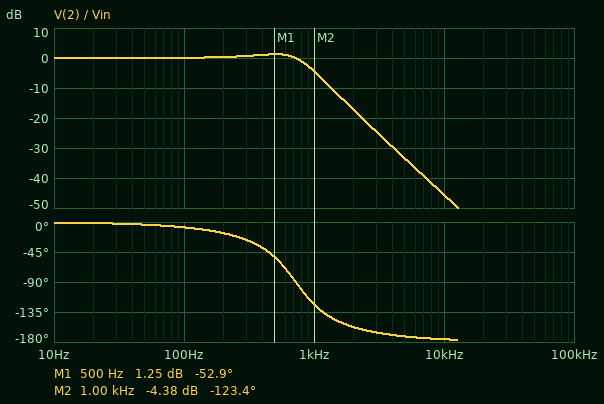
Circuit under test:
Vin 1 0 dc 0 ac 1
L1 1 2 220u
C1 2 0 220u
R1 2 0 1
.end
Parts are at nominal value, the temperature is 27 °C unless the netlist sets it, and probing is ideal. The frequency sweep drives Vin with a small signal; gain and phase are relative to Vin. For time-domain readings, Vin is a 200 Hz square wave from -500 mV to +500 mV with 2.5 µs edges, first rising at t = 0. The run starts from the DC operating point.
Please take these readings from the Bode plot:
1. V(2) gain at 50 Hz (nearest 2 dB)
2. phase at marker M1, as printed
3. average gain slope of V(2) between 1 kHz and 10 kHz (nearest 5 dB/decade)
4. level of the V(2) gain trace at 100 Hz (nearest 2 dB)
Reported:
0 dB
-52.9 deg
-40 dB/decade
0 dB
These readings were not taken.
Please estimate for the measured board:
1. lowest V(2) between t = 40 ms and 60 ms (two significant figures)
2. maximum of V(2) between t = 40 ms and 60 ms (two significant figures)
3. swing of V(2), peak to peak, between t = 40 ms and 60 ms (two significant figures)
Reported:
-660 mV
660 mV
1.3 V
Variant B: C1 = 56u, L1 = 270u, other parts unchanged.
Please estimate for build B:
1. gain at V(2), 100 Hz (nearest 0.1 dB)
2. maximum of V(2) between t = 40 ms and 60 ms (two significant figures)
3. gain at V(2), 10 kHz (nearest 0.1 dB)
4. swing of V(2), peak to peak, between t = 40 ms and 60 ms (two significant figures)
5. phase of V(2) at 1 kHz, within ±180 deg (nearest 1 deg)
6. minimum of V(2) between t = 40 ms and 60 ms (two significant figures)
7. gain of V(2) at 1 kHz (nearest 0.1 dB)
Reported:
-0.1 dB
500 mV
-35.7 dB
1.0 V
-77 deg
-500 mV
-4.8 dB
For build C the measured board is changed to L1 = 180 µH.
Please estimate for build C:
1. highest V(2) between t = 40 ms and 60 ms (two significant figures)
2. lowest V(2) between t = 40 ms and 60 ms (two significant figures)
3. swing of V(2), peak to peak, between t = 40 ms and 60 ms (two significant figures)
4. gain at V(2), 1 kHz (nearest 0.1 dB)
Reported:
700 mV
-700 mV
1.4 V
-2.0 dB
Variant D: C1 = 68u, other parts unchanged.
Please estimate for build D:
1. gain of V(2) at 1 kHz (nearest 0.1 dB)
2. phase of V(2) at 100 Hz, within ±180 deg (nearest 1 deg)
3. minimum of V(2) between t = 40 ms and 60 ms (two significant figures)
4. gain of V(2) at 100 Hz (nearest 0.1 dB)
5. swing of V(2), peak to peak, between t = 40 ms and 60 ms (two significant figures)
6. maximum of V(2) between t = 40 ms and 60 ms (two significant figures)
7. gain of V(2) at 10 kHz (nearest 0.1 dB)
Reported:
-3.2 dB
-8 deg
-500 mV
0 dB
1.0 V
500 mV
-35.5 dB
